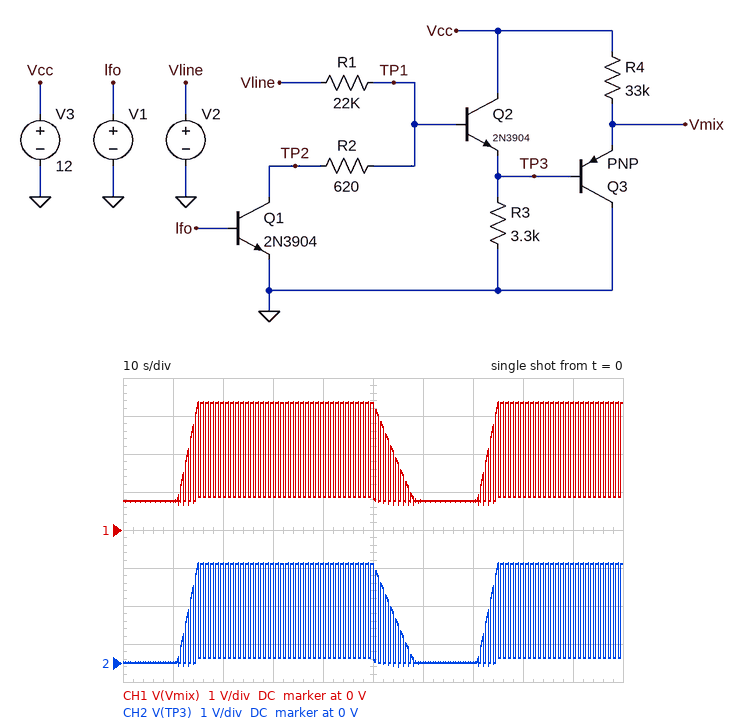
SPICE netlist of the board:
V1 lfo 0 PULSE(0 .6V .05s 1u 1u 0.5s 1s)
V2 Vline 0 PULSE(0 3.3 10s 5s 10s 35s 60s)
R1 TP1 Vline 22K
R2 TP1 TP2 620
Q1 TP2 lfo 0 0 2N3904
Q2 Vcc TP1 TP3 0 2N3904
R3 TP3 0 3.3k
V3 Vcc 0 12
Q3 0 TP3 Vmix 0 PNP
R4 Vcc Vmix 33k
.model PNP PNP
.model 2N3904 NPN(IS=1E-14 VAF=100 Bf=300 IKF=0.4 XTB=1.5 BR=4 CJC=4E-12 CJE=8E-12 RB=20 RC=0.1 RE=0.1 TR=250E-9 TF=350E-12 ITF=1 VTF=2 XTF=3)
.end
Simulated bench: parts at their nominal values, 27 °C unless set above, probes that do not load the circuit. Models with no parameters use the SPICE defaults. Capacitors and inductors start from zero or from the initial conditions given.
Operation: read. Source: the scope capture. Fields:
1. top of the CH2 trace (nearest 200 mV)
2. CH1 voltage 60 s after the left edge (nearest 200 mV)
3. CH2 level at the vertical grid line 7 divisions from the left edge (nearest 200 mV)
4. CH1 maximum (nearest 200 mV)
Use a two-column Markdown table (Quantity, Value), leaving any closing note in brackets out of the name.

| Quantity | Value |
|---|---|
| top of the CH2 trace | 2.6 V |
| CH1 voltage 60 s after the left edge | 800 mV |
| CH2 level at the vertical grid line 7 divisions from the left edge | 0 V |
| CH1 maximum | 3.4 V |
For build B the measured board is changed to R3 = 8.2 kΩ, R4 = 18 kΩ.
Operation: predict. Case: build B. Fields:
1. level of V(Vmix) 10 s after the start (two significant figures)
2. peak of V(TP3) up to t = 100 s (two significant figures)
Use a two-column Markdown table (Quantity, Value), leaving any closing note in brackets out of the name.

| Quantity | Value |
|---|---|
| level of V(Vmix) 10 s after the start | 810 mV |
| peak of V(TP3) up to t = 100 s | 2.7 V |
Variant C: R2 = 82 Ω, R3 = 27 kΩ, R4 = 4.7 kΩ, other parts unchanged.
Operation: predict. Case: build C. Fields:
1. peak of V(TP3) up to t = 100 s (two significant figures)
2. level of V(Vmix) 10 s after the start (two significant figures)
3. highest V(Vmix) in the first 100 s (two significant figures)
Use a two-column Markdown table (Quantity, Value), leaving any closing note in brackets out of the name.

| Quantity | Value |
|---|---|
| peak of V(TP3) up to t = 100 s | 2.7 V |
| level of V(Vmix) 10 s after the start | 1.4 V |
| highest V(Vmix) in the first 100 s | 3.5 V |
